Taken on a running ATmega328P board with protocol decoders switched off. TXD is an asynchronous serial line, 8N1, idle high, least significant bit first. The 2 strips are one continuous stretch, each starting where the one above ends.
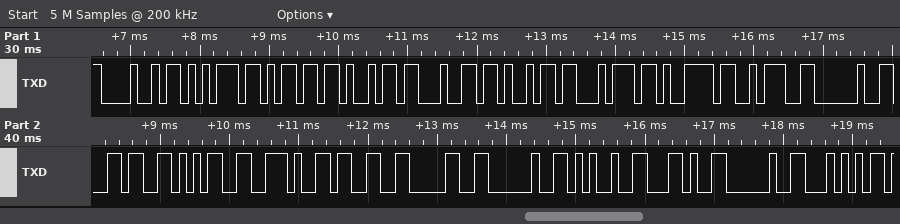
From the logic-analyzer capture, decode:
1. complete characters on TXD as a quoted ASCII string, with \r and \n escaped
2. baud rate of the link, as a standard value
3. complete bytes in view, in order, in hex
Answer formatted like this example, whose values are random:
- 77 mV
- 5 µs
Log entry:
- "Humidity: 65.30 %, T"
- 9600 baud
- 48 75 6D 69 64 69 74 79 3A 20 36 35 2E 33 30 20 25 2C 20 54
